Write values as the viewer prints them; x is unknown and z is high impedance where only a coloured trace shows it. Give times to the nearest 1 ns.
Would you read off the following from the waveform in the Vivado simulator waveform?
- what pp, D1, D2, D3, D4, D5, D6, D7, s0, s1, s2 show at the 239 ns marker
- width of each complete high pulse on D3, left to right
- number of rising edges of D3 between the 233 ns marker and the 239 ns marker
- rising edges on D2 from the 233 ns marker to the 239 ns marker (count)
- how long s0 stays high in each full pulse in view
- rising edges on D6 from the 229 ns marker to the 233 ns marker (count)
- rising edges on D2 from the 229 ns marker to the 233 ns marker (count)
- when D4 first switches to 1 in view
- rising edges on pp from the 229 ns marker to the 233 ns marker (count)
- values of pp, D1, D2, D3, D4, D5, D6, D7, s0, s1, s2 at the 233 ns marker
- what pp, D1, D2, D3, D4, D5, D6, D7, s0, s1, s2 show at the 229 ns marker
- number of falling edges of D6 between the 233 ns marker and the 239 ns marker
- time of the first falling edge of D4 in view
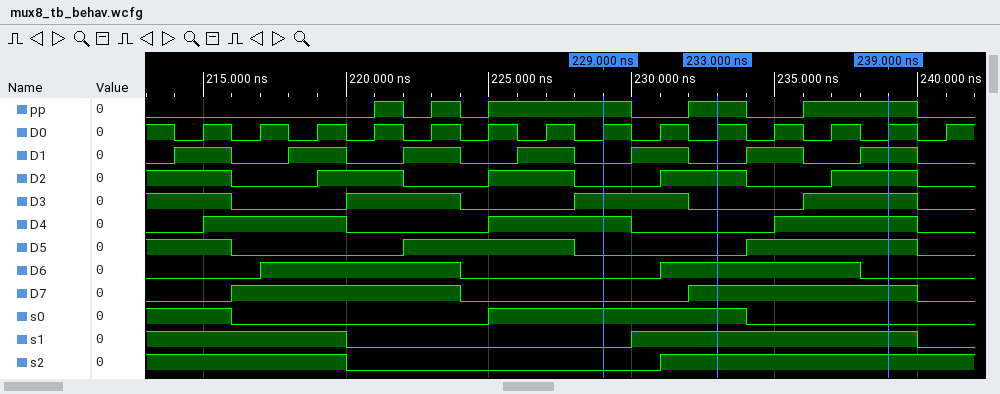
pp=1, D1=1, D2=1, D3=1, D4=1, D5=1, D6=0, D7=1, s0=0, s1=1, s2=1
4 ns, 4 ns, 4 ns
1
1
9 ns
1
1
215 ns
1
pp=1, D1=0, D2=1, D3=0, D4=0, D5=0, D6=1, D7=1, s0=1, s1=1, s2=1
pp=1, D1=0, D2=0, D3=1, D4=1, D5=0, D6=0, D7=0, s0=1, s1=0, s2=0
1
220 ns
